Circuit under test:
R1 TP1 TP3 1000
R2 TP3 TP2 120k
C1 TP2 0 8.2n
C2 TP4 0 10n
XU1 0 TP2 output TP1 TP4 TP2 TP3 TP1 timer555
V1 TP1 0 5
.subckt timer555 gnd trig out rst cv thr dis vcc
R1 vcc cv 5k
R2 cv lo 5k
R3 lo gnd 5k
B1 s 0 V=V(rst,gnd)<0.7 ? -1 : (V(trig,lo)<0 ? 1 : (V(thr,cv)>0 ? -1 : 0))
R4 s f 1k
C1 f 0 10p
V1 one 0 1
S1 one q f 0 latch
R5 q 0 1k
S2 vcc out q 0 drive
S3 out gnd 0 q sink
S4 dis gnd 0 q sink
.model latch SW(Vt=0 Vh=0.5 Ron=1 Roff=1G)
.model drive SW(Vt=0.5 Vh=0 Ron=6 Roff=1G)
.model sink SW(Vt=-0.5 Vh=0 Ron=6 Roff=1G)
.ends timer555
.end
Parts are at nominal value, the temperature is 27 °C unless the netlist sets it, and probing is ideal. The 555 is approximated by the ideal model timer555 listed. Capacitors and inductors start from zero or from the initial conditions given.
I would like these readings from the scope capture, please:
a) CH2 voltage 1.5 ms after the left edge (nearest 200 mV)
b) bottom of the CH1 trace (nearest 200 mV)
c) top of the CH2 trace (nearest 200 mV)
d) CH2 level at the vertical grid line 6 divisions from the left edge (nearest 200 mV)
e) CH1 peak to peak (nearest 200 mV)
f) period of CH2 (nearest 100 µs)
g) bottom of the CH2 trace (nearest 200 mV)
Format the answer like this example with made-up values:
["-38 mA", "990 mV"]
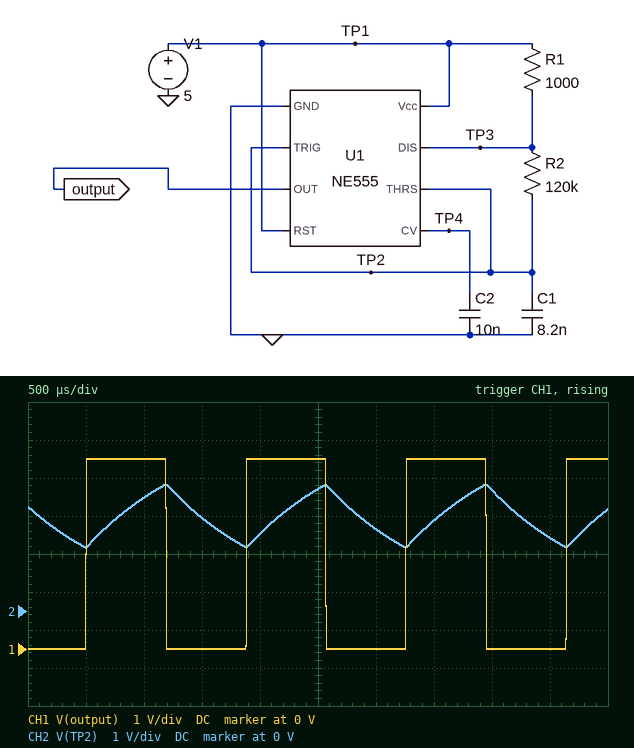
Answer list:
["2.4 V", "0 V", "3.4 V", "2.2 V", "5.0 V", "1.4 ms", "1.6 V"]
